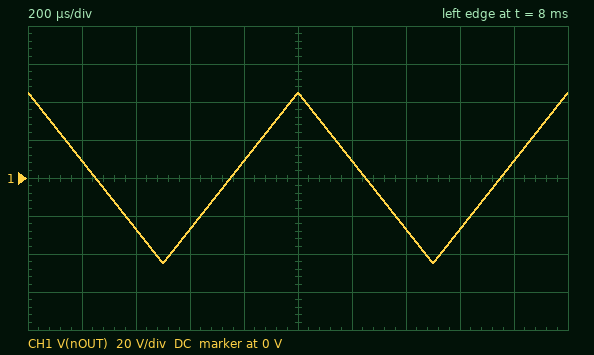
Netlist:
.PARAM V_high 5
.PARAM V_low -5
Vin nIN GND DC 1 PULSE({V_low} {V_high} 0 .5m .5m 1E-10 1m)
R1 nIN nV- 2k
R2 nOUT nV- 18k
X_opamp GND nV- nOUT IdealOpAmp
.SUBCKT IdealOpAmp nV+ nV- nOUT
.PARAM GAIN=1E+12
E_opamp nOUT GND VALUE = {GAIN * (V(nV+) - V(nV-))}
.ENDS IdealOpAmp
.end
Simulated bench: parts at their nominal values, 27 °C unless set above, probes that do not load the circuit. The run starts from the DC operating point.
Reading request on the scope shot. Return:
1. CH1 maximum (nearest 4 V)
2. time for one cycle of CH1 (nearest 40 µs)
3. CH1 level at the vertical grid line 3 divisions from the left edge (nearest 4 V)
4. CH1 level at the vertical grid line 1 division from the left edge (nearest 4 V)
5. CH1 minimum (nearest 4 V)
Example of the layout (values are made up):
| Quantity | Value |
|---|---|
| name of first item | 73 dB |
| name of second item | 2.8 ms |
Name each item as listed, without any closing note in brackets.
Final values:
| Quantity | Value |
|---|---|
| CH1 maximum | 44 V |
| time for one cycle of CH1 | 1.00 ms |
| CH1 level at the vertical grid line 3 divisions from the left edge | -28 V |
| CH1 level at the vertical grid line 1 division from the left edge | 8 V |
| CH1 minimum | -44 V |
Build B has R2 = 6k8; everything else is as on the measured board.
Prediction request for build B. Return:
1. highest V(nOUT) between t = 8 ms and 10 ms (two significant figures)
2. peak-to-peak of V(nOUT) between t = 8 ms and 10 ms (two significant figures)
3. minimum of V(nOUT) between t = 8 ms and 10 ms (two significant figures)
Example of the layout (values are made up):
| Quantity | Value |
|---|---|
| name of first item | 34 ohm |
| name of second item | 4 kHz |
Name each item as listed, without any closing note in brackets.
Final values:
| Quantity | Value |
|---|---|
| highest V(nOUT) between t = 8 ms and 10 ms | 17 V |
| peak-to-peak of V(nOUT) between t = 8 ms and 10 ms | 34 V |
| minimum of V(nOUT) between t = 8 ms and 10 ms | -17 V |
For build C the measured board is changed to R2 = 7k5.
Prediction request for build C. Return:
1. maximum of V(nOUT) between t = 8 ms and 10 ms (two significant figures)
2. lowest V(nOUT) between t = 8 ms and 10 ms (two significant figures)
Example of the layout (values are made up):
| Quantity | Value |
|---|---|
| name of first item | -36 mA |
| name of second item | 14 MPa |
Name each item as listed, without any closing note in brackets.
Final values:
| Quantity | Value |
|---|---|
| maximum of V(nOUT) between t = 8 ms and 10 ms | 19 V |
| lowest V(nOUT) between t = 8 ms and 10 ms | -19 V |
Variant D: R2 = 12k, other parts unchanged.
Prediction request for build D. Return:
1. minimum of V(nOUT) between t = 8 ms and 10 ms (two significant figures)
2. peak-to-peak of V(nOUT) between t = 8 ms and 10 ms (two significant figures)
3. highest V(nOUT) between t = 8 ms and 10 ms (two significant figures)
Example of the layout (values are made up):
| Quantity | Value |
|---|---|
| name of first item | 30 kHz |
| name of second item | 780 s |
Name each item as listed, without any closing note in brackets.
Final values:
| Quantity | Value |
|---|---|
| minimum of V(nOUT) between t = 8 ms and 10 ms | -30 V |
| peak-to-peak of V(nOUT) between t = 8 ms and 10 ms | 60 V |
| highest V(nOUT) between t = 8 ms and 10 ms | 30 V |
